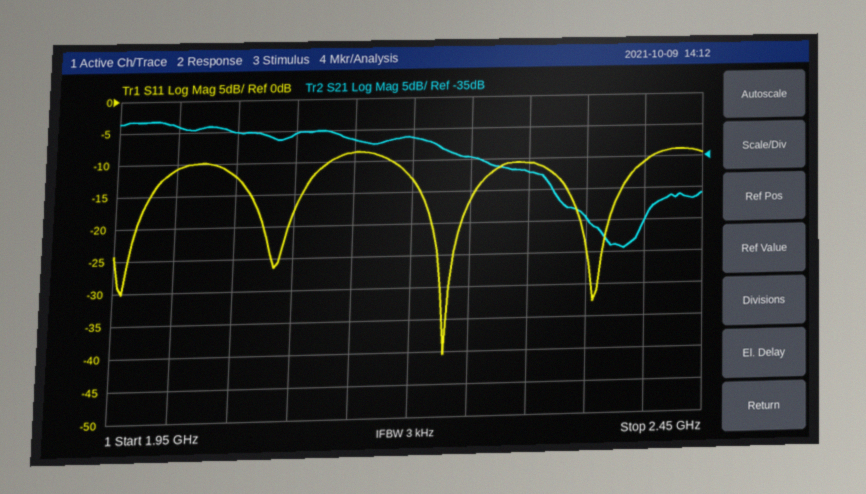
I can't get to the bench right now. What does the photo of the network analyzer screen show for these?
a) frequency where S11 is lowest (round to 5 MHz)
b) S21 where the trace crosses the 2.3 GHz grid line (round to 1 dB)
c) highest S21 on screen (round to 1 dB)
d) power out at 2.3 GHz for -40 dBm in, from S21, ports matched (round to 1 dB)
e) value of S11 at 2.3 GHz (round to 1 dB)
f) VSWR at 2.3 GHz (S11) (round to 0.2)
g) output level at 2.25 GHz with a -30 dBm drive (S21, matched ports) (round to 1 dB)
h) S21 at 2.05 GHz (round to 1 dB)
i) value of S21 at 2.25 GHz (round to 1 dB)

2.230 GHz
-37 dB
-28 dB
-77 dBm
-11 dB
1.8
-65 dBm
-30 dB
-35 dB
